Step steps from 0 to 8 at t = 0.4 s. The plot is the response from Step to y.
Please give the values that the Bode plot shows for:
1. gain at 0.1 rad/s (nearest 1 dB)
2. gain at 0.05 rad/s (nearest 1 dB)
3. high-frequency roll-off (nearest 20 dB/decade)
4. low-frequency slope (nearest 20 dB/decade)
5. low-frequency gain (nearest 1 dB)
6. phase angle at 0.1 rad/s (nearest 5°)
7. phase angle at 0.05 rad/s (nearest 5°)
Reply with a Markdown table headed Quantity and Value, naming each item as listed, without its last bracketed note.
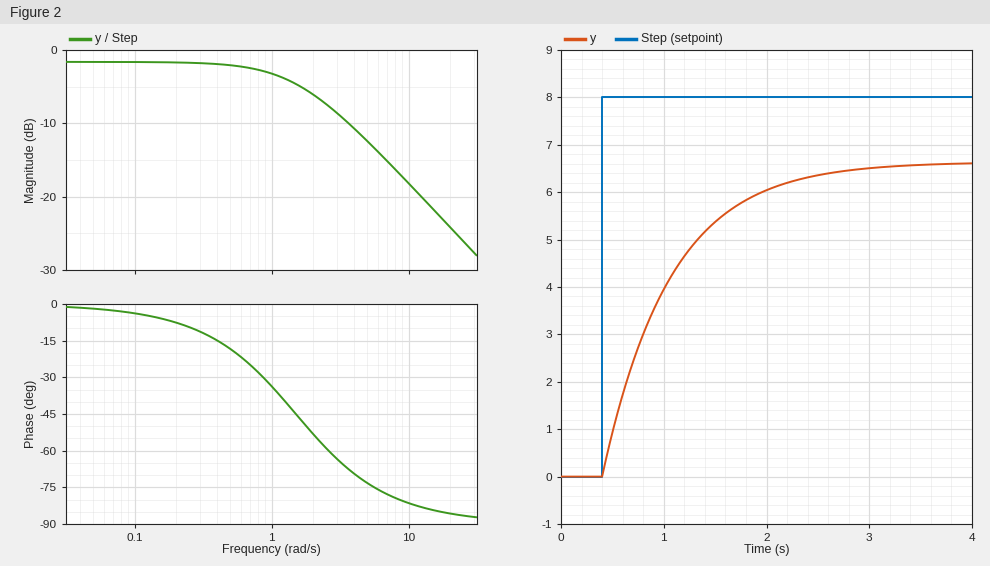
| Quantity | Value |
|---|---|
| gain at 0.1 rad/s | -2 dB |
| gain at 0.05 rad/s | -2 dB |
| high-frequency roll-off | -20 dB/decade |
| low-frequency slope | 0 dB/decade |
| low-frequency gain | -2 dB |
| phase angle at 0.1 rad/s | -5° |
| phase angle at 0.05 rad/s | 0° |
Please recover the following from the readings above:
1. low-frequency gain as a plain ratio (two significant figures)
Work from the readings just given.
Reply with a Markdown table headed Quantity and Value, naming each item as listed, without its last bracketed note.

| Quantity | Value |
|---|---|
| low-frequency gain as a plain ratio | 0.79 |
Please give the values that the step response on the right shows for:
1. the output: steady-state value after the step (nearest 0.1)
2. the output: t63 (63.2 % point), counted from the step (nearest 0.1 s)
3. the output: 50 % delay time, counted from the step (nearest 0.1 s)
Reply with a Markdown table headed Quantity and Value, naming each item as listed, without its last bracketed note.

| Quantity | Value |
|---|---|
| the output: steady-state value after the step | 6.6 |
| the output: t63 (63.2 % point), counted from the step | 0.7 s |
| the output: 50 % delay time, counted from the step | 0.5 s |
